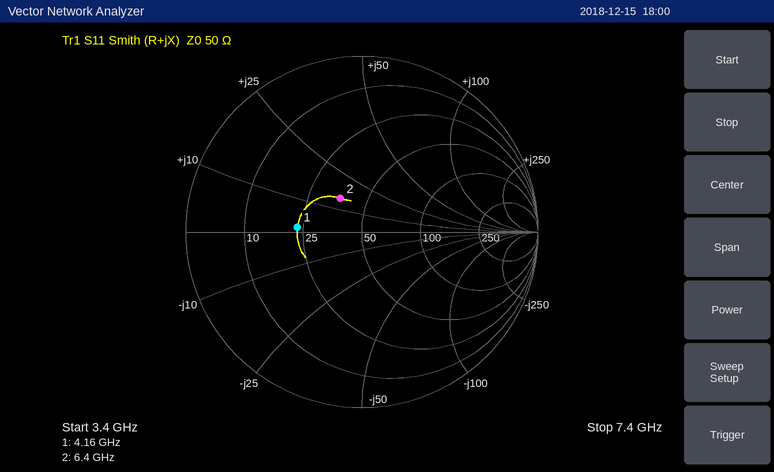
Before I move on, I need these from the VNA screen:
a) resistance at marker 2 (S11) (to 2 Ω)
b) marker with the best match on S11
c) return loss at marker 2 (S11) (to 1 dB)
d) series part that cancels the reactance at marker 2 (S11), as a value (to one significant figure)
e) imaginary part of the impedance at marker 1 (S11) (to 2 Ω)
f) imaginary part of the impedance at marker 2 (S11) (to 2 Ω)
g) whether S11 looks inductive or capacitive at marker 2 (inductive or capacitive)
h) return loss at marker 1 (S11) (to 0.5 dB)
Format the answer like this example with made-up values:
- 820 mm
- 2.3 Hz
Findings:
- 36 Ω
- marker 2
- 13 dB
- 2 pF
- +2 Ω
- +14 Ω
- inductive
- 8.5 dB
